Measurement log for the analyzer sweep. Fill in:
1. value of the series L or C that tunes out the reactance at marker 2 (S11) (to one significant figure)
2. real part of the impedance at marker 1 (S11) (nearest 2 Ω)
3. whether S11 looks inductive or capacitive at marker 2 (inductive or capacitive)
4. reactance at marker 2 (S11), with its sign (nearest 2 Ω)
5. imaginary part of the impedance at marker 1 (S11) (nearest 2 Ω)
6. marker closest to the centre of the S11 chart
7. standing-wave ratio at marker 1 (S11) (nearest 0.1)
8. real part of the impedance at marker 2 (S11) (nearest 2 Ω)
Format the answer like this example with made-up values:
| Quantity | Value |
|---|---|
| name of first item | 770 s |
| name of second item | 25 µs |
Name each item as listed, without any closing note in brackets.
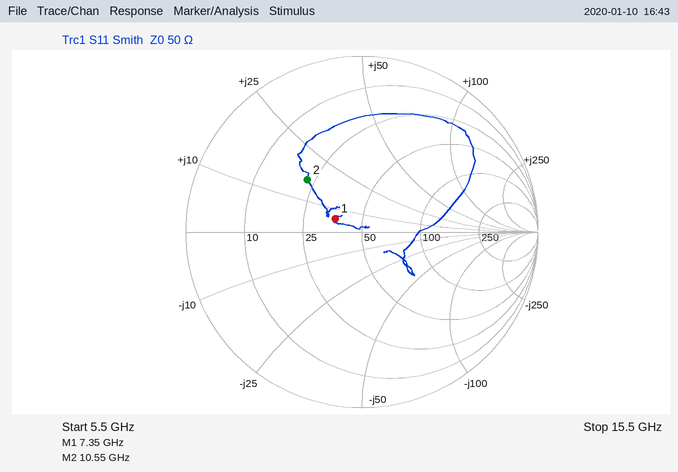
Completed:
| Quantity | Value |
|---|---|
| value of the series L or C that tunes out the reactance at marker 2 (S11) | 900 fF |
| real part of the impedance at marker 1 (S11) | 36 Ω |
| whether S11 looks inductive or capacitive at marker 2 | inductive |
| reactance at marker 2 (S11), with its sign | +16 Ω |
| imaginary part of the impedance at marker 1 (S11) | +6 Ω |
| marker closest to the centre of the S11 chart | marker 1 |
| standing-wave ratio at marker 1 (S11) | 1.4 |
| real part of the impedance at marker 2 (S11) | 22 Ω |
